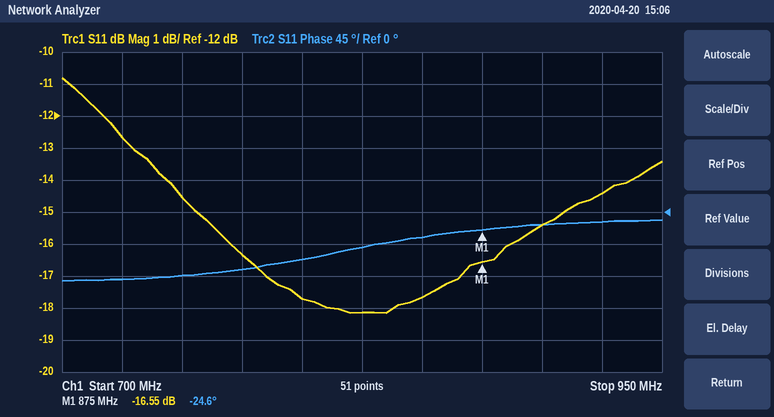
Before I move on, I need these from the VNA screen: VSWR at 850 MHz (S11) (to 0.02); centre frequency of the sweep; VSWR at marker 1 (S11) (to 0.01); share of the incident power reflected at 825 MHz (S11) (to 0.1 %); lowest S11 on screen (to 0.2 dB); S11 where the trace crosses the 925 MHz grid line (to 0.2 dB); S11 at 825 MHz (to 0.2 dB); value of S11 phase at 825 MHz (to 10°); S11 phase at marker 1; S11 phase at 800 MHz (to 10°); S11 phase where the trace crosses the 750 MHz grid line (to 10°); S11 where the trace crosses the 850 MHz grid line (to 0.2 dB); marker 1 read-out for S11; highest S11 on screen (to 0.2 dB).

1.30
825 MHz
1.35
1.5 %
-18.2 dB
-14.4 dB
-18.2 dB
-50°
-24.6°
-70°
-90°
-17.6 dB
-16.55 dB
-10.8 dB
